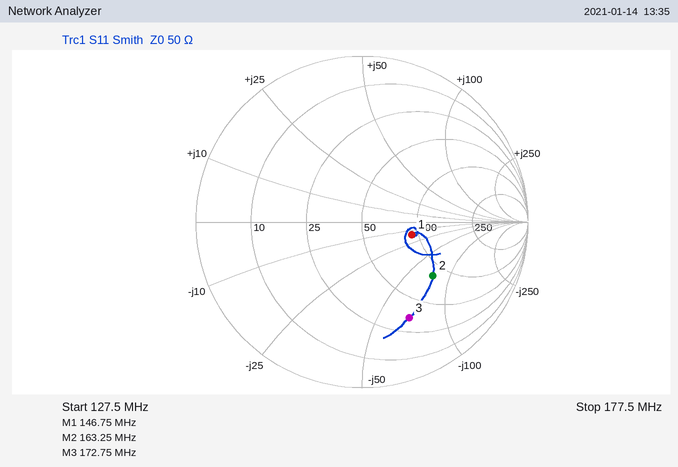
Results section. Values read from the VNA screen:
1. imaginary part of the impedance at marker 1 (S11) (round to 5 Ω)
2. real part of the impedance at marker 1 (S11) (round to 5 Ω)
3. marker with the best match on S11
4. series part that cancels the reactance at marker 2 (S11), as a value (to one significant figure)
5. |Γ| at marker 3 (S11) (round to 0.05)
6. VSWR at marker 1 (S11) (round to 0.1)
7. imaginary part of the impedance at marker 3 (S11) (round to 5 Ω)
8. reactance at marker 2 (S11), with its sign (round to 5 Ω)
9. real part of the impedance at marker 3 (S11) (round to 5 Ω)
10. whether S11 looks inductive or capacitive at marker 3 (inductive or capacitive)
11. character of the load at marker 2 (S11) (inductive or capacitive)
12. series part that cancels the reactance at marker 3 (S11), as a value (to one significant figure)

-15 Ω
90 Ω
marker 1
70 nH
0.65
1.9
-70 Ω
-75 Ω
35 Ω
capacitive
capacitive
60 nH
